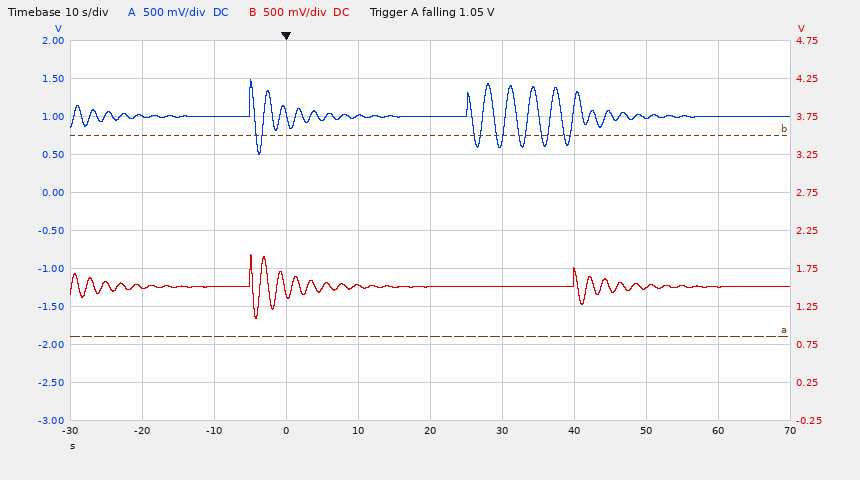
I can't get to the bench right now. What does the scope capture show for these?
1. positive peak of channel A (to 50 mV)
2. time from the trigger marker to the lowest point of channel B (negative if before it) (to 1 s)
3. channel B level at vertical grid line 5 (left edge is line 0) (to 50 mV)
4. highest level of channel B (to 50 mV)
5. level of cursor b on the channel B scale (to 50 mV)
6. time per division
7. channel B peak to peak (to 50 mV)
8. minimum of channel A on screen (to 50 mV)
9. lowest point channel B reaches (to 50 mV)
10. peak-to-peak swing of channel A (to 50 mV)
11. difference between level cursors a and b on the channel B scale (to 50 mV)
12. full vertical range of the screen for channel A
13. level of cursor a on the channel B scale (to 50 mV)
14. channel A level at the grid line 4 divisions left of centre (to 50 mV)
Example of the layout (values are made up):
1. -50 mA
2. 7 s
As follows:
1. 1.50 V
2. -4 s
3. 1.50 V
4. 1.95 V
5. 3.50 V
6. 10 s
7. 850 mV
8. 500 mV
9. 1.10 V
10. 1.00 V
11. 2.65 V
12. 5 V
13. 850 mV
14. 1.00 V
